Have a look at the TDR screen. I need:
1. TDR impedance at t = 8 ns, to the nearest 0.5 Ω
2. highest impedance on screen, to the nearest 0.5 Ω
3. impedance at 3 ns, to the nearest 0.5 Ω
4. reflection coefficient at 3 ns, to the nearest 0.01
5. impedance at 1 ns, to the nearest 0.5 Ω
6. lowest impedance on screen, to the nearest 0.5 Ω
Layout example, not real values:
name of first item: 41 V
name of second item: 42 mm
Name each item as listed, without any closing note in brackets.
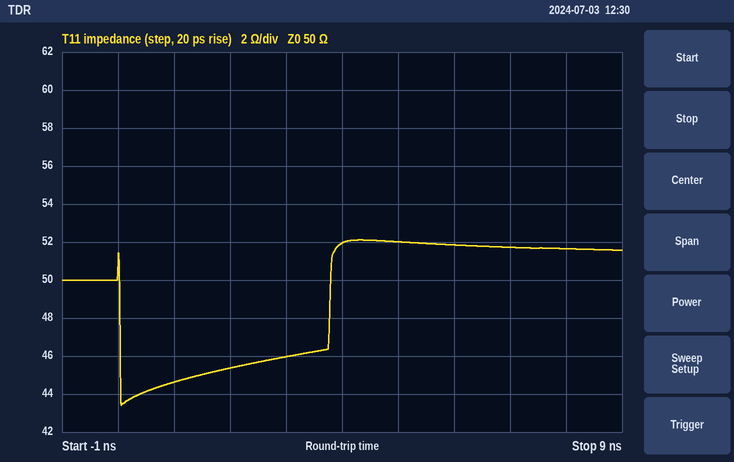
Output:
TDR impedance at t = 8 ns, to the nearest 0.5 Ω: 51.5 Ω
highest impedance on screen, to the nearest 0.5 Ω: 52.0 Ω
impedance at 3 ns, to the nearest 0.5 Ω: 46.0 Ω
reflection coefficient at 3 ns, to the nearest 0.01: -0.04
impedance at 1 ns, to the nearest 0.5 Ω: 44.5 Ω
lowest impedance on screen, to the nearest 0.5 Ω: 43.5 Ω
